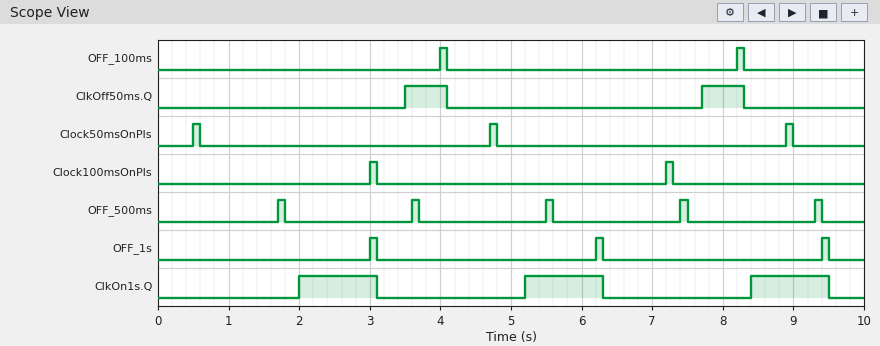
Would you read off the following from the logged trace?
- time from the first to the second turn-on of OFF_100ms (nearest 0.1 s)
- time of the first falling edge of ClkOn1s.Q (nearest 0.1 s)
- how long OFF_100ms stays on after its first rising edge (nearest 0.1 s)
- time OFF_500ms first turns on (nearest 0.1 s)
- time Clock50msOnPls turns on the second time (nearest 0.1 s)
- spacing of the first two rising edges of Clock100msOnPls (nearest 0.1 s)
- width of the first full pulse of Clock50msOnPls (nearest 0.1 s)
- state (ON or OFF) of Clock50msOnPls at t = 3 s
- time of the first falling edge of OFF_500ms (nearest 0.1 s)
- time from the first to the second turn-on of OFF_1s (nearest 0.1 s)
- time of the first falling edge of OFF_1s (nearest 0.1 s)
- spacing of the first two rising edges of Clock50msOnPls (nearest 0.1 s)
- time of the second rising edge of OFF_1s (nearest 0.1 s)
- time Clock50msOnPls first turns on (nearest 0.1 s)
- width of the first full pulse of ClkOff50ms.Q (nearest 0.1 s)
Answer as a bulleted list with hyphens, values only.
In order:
- 4.2 s
- 3.1 s
- 0.1 s
- 1.7 s
- 4.7 s
- 4.2 s
- 0.1 s
- OFF
- 1.8 s
- 3.2 s
- 3.1 s
- 4.2 s
- 6.2 s
- 0.5 s
- 0.6 s
